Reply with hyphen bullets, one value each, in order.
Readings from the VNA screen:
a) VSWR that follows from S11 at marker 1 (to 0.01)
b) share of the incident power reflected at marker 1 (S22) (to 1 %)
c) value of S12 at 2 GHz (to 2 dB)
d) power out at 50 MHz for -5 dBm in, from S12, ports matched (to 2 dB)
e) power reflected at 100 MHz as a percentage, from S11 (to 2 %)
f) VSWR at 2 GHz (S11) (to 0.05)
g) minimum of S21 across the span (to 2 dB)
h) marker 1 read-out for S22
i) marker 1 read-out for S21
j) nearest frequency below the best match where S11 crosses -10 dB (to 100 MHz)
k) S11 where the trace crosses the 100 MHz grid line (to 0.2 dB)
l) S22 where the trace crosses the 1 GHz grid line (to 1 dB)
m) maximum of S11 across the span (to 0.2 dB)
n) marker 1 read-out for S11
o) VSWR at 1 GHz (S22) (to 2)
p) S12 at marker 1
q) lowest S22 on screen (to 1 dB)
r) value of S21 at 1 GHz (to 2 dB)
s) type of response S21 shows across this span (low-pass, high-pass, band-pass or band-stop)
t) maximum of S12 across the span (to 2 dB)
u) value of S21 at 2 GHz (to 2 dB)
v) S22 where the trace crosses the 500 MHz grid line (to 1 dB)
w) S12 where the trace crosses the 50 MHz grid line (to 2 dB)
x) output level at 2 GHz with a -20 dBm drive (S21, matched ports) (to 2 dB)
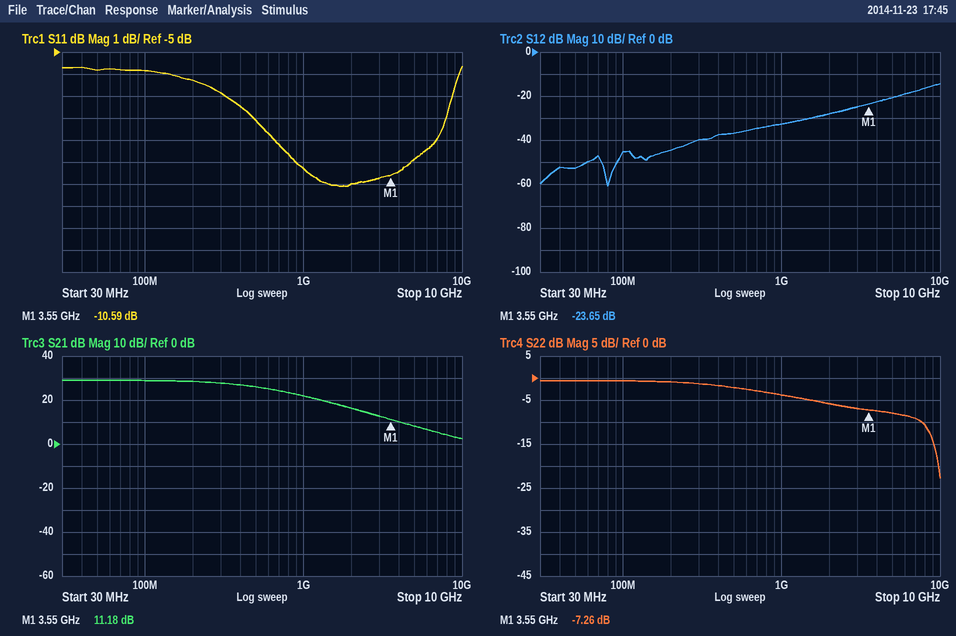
- 1.84
- 19 %
- -28 dB
- -58 dBm
- 26 %
- 1.80
- 2 dB
- -7.26 dB
- 11.18 dB
- 900 MHz
- -5.8 dB
- -4 dB
- -5.6 dB
- -10.59 dB
- 4
- -23.65 dB
- -23 dB
- 22 dB
- low-pass
- -14 dB
- 16 dB
- -2 dB
- -52 dB
- -4 dBm
